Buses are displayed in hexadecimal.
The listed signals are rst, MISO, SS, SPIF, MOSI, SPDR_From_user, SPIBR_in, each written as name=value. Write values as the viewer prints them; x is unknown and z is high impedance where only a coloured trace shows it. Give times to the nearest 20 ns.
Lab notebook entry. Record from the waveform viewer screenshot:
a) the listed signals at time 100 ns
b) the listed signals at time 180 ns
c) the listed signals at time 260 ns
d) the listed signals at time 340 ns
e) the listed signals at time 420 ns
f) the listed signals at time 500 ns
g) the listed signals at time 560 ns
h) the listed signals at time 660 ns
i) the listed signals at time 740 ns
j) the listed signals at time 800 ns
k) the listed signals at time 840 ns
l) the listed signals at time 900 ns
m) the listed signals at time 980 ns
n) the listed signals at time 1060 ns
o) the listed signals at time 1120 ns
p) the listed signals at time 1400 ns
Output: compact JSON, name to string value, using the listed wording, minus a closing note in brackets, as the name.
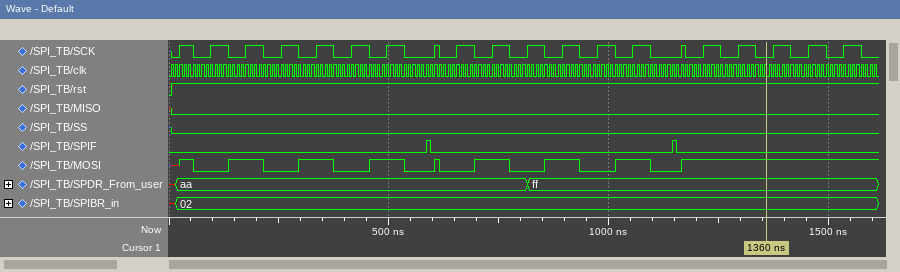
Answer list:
{"the listed signals at time 100 ns": "rst=1, MISO=0, SS=0, SPIF=0, MOSI=0, SPDR_From_user=aa, SPIBR_in=02", "the listed signals at time 180 ns": "rst=1, MISO=0, SS=0, SPIF=0, MOSI=1, SPDR_From_user=aa, SPIBR_in=02", "the listed signals at time 260 ns": "rst=1, MISO=0, SS=0, SPIF=0, MOSI=0, SPDR_From_user=aa, SPIBR_in=02", "the listed signals at time 340 ns": "rst=1, MISO=0, SS=0, SPIF=0, MOSI=1, SPDR_From_user=aa, SPIBR_in=02", "the listed signals at time 420 ns": "rst=1, MISO=0, SS=0, SPIF=0, MOSI=0, SPDR_From_user=aa, SPIBR_in=02", "the listed signals at time 500 ns": "rst=1, MISO=0, SS=0, SPIF=0, MOSI=1, SPDR_From_user=aa, SPIBR_in=02", "the listed signals at time 560 ns": "rst=1, MISO=0, SS=0, SPIF=0, MOSI=0, SPDR_From_user=aa, SPIBR_in=02", "the listed signals at time 660 ns": "rst=1, MISO=0, SS=0, SPIF=0, MOSI=0, SPDR_From_user=aa, SPIBR_in=02", "the listed signals at time 740 ns": "rst=1, MISO=0, SS=0, SPIF=0, MOSI=1, SPDR_From_user=aa, SPIBR_in=02", "the listed signals at time 800 ns": "rst=1, MISO=0, SS=0, SPIF=0, MOSI=0, SPDR_From_user=aa, SPIBR_in=02", "the listed signals at time 840 ns": "rst=1, MISO=0, SS=0, SPIF=0, MOSI=0, SPDR_From_user=ff, SPIBR_in=02", "the listed signals at time 900 ns": "rst=1, MISO=0, SS=0, SPIF=0, MOSI=1, SPDR_From_user=ff, SPIBR_in=02", "the listed signals at time 980 ns": "rst=1, MISO=0, SS=0, SPIF=0, MOSI=0, SPDR_From_user=ff, SPIBR_in=02", "the listed signals at time 1060 ns": "rst=1, MISO=0, SS=0, SPIF=0, MOSI=1, SPDR_From_user=ff, SPIBR_in=02", "the listed signals at time 1120 ns": "rst=1, MISO=0, SS=0, SPIF=0, MOSI=0, SPDR_From_user=ff, SPIBR_in=02", "the listed signals at time 1400 ns": "rst=1, MISO=0, SS=0, SPIF=0, MOSI=1, SPDR_From_user=ff, SPIBR_in=02"}
